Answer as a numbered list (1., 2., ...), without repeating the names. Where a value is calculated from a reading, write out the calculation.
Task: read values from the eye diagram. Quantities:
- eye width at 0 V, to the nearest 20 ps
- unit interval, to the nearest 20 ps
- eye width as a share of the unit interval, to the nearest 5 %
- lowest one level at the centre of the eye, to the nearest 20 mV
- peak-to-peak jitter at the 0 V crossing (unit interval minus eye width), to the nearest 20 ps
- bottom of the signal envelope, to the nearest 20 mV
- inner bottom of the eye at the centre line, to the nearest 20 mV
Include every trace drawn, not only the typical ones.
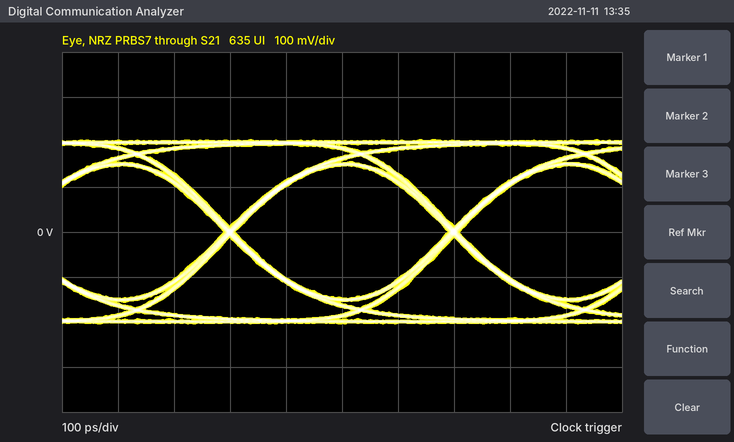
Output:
1. 380 ps
2. 400 ps
3. 380 ps / 400 ps ≈ 95 %
4. 140 mV
5. 20 ps
6. -200 mV
7. -140 mV
